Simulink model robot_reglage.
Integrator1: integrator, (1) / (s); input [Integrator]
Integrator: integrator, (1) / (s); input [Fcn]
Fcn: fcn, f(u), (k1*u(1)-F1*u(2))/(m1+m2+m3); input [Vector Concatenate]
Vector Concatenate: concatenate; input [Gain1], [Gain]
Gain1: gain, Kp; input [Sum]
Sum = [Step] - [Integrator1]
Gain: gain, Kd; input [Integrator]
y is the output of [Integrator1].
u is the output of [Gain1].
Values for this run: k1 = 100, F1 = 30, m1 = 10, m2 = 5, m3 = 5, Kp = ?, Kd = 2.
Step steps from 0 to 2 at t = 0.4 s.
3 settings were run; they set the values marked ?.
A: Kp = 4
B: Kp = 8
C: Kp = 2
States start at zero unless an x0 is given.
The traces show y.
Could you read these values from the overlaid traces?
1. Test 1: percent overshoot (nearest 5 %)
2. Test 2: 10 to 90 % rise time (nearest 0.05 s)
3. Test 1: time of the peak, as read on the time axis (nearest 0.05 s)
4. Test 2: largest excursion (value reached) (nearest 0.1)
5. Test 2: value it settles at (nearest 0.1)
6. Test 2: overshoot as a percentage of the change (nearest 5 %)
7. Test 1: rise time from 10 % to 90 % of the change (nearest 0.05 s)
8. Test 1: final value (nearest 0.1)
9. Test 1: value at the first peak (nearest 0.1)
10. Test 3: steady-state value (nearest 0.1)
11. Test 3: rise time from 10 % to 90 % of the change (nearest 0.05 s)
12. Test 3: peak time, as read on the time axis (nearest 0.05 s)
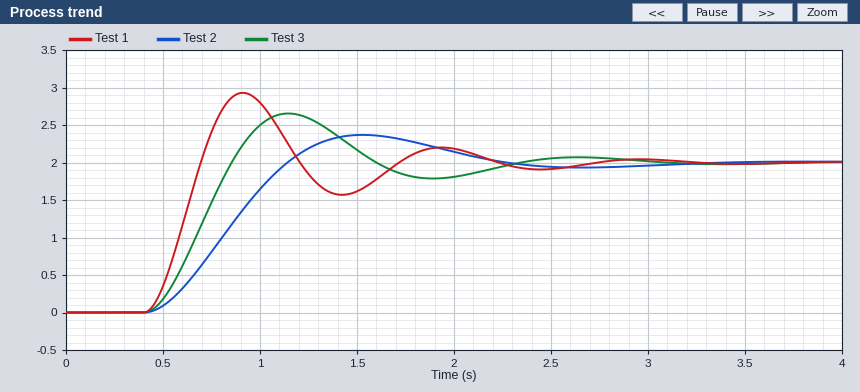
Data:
45 %
0.50 s
0.90 s
2.4
2.0
20 %
0.20 s
2.0
2.9
2.0
0.30 s
1.15 s
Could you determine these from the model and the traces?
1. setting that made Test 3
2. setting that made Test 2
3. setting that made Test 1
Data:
A
C
B
